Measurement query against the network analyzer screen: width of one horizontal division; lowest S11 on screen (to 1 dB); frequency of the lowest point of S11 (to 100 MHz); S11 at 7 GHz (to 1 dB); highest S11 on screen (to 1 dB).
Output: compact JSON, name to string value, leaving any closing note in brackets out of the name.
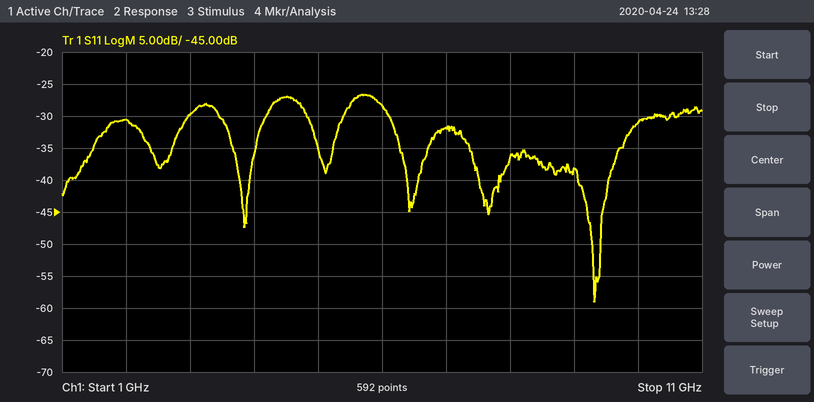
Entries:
{"width of one horizontal division": "1 GHz", "lowest S11 on screen": "-59 dB", "frequency of the lowest point of S11": "9.3 GHz", "S11 at 7 GHz": "-32 dB", "highest S11 on screen": "-27 dB"}
